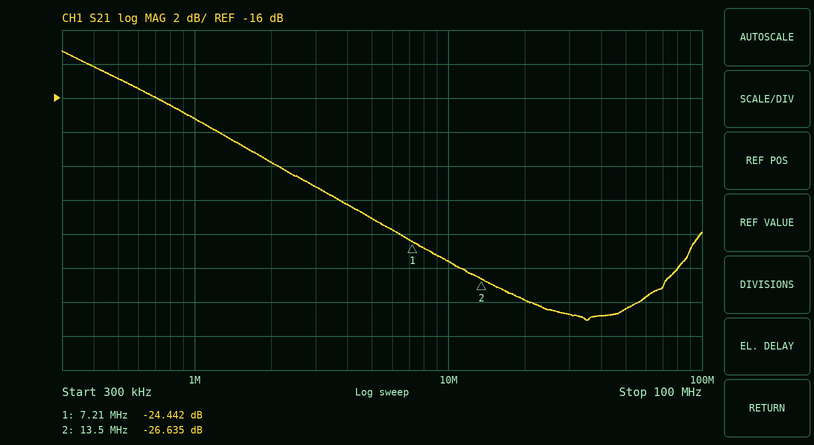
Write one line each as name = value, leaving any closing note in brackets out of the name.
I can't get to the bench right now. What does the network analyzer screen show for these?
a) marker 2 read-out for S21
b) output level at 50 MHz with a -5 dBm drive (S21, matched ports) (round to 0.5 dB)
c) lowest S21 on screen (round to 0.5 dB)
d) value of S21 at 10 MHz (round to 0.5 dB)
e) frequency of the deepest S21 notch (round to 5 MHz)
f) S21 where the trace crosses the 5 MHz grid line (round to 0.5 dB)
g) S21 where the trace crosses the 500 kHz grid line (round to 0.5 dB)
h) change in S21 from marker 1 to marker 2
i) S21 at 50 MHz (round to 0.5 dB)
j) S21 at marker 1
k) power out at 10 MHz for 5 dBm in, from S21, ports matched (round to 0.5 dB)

marker 2 read-out for S21 = -26.635 dB
output level at 50 MHz with a -5 dBm drive (S21, matched ports) = -33.5 dBm
lowest S21 on screen = -29.0 dB
value of S21 at 10 MHz = -25.5 dB
frequency of the deepest S21 notch = 35 MHz
S21 where the trace crosses the 5 MHz grid line = -23.0 dB
S21 where the trace crosses the 500 kHz grid line = -15.0 dB
change in S21 from marker 1 to marker 2 = -2.193 dB
S21 at 50 MHz = -28.5 dB
S21 at marker 1 = -24.442 dB
power out at 10 MHz for 5 dBm in, from S21, ports matched = -20.5 dBm
